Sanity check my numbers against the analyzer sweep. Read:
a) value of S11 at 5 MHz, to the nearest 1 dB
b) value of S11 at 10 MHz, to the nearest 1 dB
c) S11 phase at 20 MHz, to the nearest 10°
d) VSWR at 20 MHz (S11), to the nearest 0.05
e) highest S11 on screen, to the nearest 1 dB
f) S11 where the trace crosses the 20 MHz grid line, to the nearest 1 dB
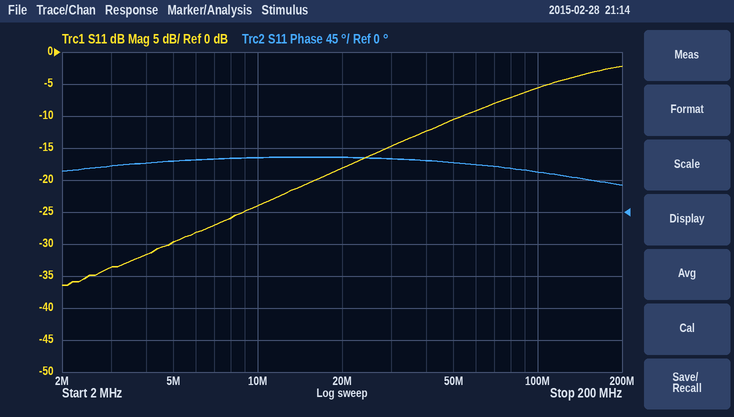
-30 dB
-24 dB
80°
1.30
-2 dB
-18 dB
